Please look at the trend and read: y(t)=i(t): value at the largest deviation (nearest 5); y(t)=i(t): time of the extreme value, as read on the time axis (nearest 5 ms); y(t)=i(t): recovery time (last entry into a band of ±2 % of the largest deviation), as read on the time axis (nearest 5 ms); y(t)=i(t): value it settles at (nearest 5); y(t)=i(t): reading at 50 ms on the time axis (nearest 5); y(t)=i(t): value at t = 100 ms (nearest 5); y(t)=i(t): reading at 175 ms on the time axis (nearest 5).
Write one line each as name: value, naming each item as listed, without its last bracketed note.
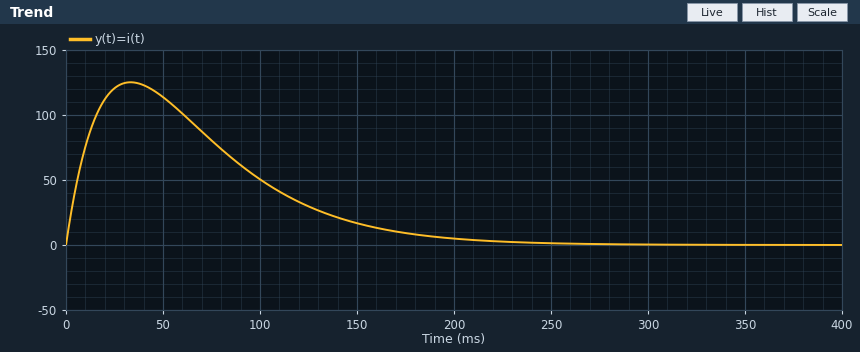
y(t)=i(t): value at the largest deviation: 125
y(t)=i(t): time of the extreme value, as read on the time axis: 35 ms
y(t)=i(t): recovery time (last entry into a band of ±2 % of the largest deviation), as read on the time axis: 225 ms
y(t)=i(t): value it settles at: 0
y(t)=i(t): reading at 50 ms on the time axis: 115
y(t)=i(t): value at t = 100 ms: 50
y(t)=i(t): reading at 175 ms on the time axis: 10
